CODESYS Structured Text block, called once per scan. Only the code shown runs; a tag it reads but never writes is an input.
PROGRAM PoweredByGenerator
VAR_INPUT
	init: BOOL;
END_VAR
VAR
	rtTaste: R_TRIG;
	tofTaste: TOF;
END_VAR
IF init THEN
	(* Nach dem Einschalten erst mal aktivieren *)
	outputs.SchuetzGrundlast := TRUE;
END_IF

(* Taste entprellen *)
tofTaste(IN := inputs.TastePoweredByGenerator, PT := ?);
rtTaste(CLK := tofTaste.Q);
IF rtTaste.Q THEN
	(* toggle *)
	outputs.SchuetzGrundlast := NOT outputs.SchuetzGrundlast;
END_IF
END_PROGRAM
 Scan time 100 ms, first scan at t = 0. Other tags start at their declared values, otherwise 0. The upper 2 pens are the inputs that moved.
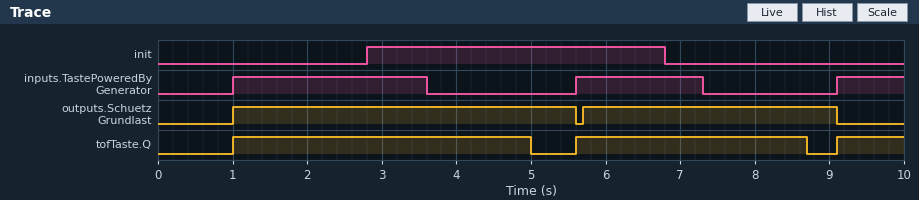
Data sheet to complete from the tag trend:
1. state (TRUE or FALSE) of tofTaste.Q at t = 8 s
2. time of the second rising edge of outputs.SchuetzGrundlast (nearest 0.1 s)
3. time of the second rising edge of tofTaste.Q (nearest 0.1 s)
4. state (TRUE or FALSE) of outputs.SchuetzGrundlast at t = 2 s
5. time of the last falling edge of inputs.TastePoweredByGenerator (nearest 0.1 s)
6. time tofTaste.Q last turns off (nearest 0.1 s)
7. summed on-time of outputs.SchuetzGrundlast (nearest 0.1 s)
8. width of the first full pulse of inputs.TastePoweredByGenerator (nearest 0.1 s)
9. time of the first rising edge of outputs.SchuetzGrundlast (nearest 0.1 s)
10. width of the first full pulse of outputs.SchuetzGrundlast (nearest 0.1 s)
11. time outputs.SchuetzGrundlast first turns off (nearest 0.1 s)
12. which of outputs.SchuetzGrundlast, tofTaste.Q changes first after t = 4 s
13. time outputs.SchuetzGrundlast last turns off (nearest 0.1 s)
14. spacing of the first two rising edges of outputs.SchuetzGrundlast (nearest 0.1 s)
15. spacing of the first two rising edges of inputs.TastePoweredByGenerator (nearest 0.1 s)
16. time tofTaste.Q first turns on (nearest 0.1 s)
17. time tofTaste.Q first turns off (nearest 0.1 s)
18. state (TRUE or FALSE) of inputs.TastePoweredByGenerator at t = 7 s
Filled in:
TRUE
5.7 s
5.6 s
TRUE
7.3 s
8.7 s
8.0 s
2.6 s
1.0 s
4.6 s
5.6 s
tofTaste.Q
9.1 s
4.7 s
4.6 s
1.0 s
5.0 s
TRUE
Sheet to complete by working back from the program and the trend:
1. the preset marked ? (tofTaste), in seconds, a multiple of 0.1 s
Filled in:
1.4 s
